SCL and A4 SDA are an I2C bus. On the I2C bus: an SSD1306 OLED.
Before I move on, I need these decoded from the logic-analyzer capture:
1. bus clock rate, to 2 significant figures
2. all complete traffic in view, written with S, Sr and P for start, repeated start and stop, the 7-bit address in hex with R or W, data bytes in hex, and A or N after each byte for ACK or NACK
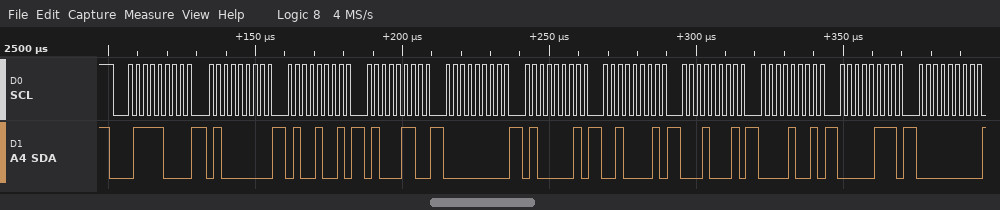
400 kHz
S 3CW A 40 A 49 A 46 A 00 A 41 A 21 A 11 A 09 A 07 A 00 A
